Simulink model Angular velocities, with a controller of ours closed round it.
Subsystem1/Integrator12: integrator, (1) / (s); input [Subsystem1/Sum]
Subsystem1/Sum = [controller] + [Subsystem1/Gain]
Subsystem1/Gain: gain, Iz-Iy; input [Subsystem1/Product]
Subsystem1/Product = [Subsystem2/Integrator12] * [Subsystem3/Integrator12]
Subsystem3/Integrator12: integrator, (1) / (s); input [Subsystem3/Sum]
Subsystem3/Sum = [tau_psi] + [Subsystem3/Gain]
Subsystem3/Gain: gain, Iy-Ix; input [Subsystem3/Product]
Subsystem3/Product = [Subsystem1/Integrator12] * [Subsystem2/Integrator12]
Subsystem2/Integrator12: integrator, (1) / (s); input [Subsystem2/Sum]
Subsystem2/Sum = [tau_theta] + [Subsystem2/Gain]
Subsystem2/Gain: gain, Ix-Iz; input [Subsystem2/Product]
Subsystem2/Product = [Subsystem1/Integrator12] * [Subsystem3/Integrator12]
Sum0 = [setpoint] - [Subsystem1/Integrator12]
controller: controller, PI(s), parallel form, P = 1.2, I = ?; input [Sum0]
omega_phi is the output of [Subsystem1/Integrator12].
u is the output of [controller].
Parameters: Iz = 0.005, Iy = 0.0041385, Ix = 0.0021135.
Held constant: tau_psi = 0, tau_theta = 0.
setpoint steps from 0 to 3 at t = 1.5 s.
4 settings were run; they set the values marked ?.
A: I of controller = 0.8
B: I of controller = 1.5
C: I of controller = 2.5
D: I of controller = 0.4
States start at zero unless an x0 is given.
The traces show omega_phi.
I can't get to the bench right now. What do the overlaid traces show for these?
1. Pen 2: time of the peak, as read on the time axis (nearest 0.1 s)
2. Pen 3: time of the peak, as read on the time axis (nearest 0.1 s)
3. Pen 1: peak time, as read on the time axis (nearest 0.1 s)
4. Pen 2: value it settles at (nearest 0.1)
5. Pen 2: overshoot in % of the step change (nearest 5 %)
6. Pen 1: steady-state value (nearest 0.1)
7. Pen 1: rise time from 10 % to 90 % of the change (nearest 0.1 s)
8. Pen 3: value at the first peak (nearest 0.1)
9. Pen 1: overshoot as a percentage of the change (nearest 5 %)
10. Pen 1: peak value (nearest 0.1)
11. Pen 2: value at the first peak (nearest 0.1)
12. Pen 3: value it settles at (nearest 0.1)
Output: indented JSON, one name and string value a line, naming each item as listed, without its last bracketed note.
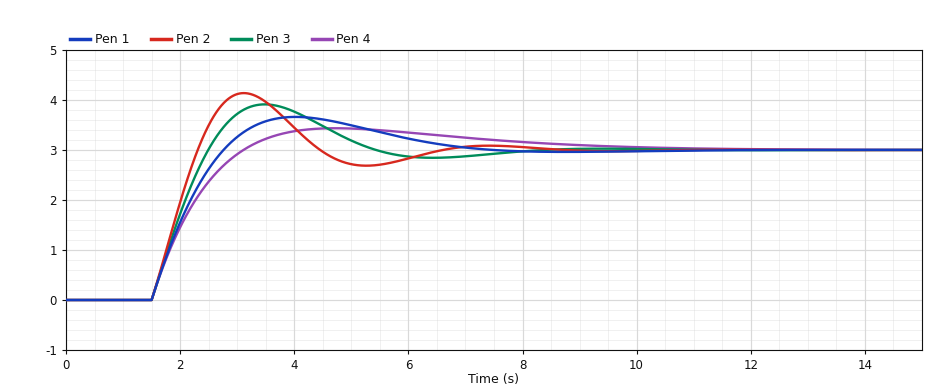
{
  "Pen 2: time of the peak, as read on the time axis": "3.1 s",
  "Pen 3: time of the peak, as read on the time axis": "3.5 s",
  "Pen 1: peak time, as read on the time axis": "4.0 s",
  "Pen 2: value it settles at": "3.0",
  "Pen 2: overshoot in % of the step change": "40 %",
  "Pen 1: steady-state value": "3.0",
  "Pen 1: rise time from 10 % to 90 % of the change": "1.0 s",
  "Pen 3: value at the first peak": "3.9",
  "Pen 1: overshoot as a percentage of the change": "20 %",
  "Pen 1: peak value": "3.7",
  "Pen 2: value at the first peak": "4.1",
  "Pen 3: value it settles at": "3.0"
}
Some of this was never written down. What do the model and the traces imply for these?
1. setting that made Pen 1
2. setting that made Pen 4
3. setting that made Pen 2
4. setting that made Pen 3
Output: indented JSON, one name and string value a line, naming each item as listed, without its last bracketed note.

{
  "setting that made Pen 1": "A",
  "setting that made Pen 4": "D",
  "setting that made Pen 2": "C",
  "setting that made Pen 3": "B"
}
